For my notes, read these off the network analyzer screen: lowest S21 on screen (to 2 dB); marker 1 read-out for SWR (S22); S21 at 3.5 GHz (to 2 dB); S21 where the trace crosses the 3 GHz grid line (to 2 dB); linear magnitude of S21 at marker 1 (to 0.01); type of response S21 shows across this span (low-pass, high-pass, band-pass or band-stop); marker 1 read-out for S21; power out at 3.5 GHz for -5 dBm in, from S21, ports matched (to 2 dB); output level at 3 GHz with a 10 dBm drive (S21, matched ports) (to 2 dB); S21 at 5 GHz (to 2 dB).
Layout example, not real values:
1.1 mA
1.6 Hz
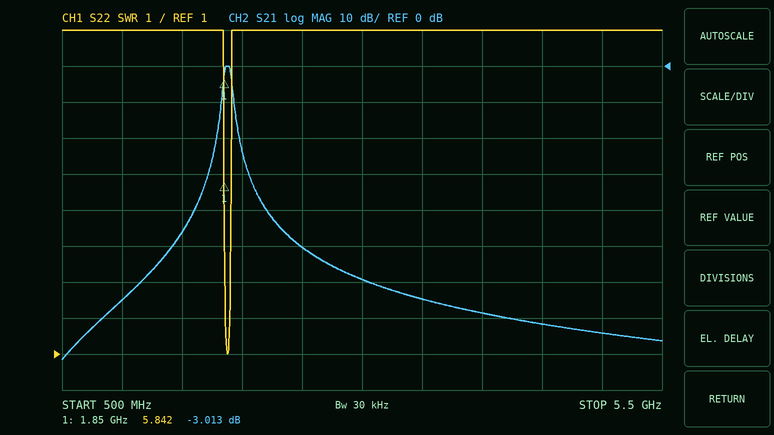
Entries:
-82 dB
5.842
-64 dB
-60 dB
0.71
band-pass
-3.013 dB
-70 dBm
-50 dBm
-74 dB
